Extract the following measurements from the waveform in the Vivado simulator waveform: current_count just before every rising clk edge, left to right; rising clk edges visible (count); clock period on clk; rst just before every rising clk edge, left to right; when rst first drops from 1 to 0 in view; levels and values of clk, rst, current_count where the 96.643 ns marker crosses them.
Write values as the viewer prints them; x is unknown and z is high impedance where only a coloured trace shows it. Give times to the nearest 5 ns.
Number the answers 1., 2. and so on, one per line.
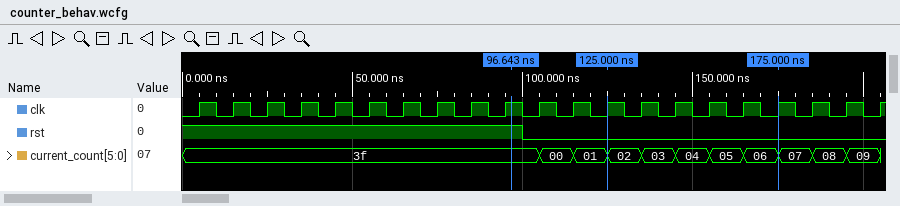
1. 3f, 3f, 3f, 3f, 3f, 3f, 3f, 3f, 3f, 3f, 3f, 00, 01, 02, 03, 04, 05, 06, 07, 08, 09
2. 21
3. 10 ns
4. 1 1 1 1 1 1 1 1 1 1 0 0 0 0 0 0 0 0 0 0 0
5. 100 ns
6. clk=1, rst=1, current_count=3f
